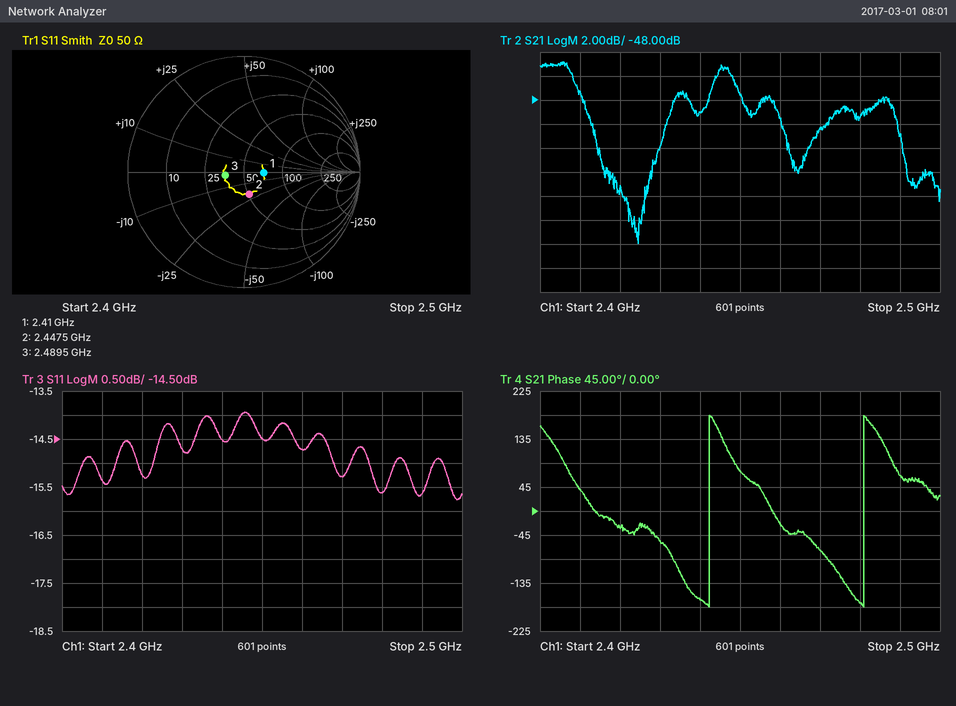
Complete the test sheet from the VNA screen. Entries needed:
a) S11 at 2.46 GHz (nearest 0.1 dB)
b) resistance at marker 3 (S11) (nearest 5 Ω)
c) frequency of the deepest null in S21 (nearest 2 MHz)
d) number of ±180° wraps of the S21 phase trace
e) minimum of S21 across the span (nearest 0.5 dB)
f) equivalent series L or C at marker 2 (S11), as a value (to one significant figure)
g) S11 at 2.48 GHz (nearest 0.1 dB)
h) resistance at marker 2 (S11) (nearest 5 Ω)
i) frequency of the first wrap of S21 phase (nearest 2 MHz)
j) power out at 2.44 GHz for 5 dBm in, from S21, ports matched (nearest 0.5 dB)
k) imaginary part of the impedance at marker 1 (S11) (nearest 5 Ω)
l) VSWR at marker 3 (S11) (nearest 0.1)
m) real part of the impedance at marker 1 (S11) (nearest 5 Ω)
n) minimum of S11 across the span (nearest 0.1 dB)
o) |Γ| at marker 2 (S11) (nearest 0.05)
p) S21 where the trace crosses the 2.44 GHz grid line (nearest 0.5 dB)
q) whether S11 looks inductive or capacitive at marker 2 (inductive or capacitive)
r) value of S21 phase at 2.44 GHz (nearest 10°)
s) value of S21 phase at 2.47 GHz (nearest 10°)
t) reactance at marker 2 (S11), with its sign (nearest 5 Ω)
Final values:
-14.7 dB
35 Ω
2.424 GHz
2
-60.0 dB
3 pF
-15.6 dB
50 Ω
2.442 GHz
-44.0 dBm
0 Ω
1.4
70 Ω
-15.8 dB
0.20
-49.0 dB
capacitive
-170°
-70°
-20 Ω
